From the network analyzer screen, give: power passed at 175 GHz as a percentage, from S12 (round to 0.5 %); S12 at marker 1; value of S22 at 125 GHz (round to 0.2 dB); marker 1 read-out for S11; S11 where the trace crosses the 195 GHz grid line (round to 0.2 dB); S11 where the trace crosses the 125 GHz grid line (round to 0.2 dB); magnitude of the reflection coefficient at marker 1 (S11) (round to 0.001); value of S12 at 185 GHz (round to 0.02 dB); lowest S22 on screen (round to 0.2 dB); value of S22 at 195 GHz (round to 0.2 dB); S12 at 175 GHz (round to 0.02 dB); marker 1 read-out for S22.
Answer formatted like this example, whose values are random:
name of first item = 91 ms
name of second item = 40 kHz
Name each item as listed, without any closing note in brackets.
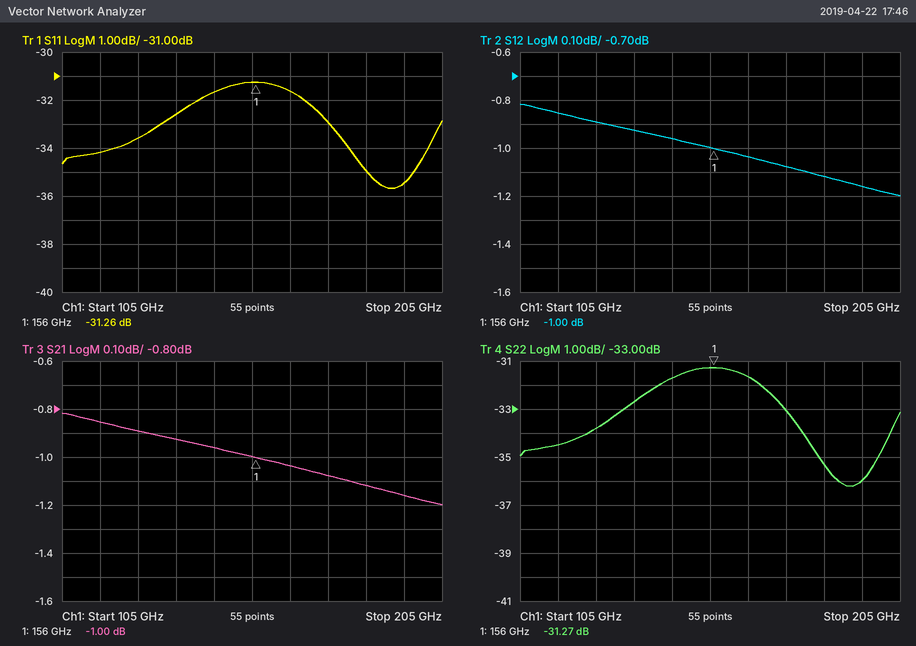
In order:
power passed at 175 GHz as a percentage, from S12 = 78.0 %
S12 at marker 1 = -1.00 dB
value of S22 at 125 GHz = -33.8 dB
marker 1 read-out for S11 = -31.26 dB
S11 where the trace crosses the 195 GHz grid line = -35.4 dB
S11 where the trace crosses the 125 GHz grid line = -33.6 dB
magnitude of the reflection coefficient at marker 1 (S11) = 0.027
value of S12 at 185 GHz = -1.12 dB
lowest S22 on screen = -36.2 dB
value of S22 at 195 GHz = -36.0 dB
S12 at 175 GHz = -1.08 dB
marker 1 read-out for S22 = -31.27 dB
